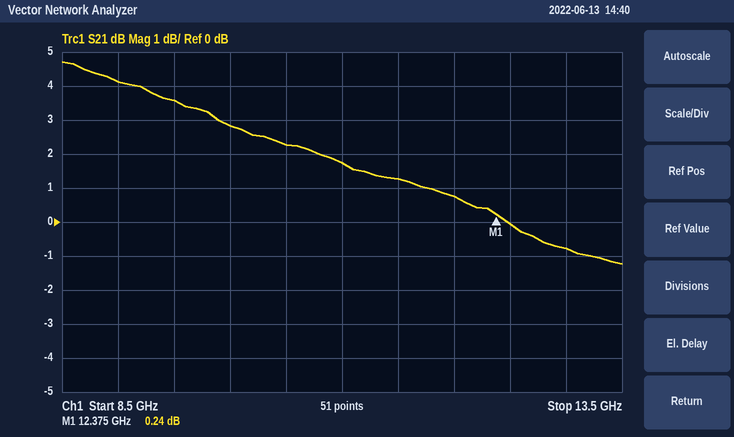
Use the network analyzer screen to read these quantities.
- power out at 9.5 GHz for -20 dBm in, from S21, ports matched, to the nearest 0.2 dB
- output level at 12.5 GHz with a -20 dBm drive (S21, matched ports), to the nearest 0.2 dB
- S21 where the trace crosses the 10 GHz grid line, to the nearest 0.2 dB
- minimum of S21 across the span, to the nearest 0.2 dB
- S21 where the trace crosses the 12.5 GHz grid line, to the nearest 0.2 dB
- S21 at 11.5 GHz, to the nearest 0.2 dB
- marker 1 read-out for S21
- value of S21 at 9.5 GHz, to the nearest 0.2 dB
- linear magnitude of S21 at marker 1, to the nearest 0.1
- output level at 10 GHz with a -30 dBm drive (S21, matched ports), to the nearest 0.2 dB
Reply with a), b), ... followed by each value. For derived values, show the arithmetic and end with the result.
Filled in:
a) -20 dBm + (3.6 dB) = -16.4 dBm
b) -20 dBm + (0.0 dB) = -20.0 dBm
c) 2.8 dB
d) -1.2 dB
e) 0.0 dB
f) 1.2 dB
g) 0.24 dB
h) 3.6 dB
i) 10^(0.24/20) ≈ 1.0
j) -30 dBm + (2.8 dB) = -27.2 dBm
